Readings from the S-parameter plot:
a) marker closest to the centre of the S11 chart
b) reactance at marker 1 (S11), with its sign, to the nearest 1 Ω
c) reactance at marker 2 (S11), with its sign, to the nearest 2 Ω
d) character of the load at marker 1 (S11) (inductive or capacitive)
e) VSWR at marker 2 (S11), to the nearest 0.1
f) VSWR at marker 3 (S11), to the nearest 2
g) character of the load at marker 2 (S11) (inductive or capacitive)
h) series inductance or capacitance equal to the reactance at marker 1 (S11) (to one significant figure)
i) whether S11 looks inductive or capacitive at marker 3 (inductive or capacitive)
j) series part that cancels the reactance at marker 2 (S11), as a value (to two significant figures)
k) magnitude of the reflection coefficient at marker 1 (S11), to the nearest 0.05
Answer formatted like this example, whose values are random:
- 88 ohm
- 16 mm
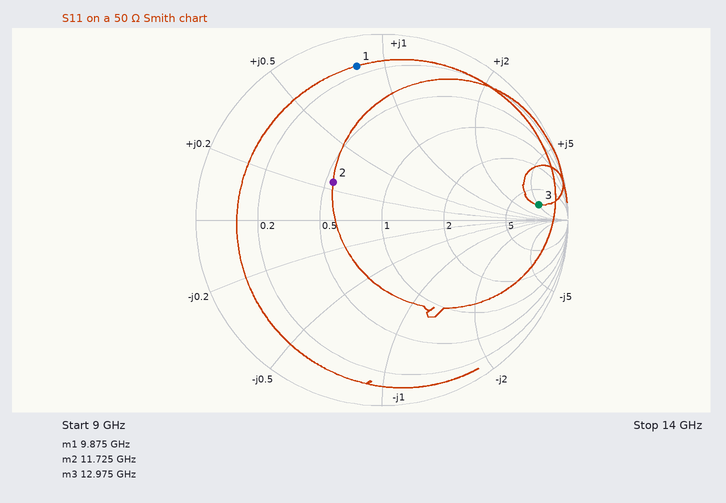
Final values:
- marker 2
- +42 Ω
- +12 Ω
- inductive
- 2.0
- 12
- inductive
- 700 pH
- inductive
- 1.1 pF
- 0.85
